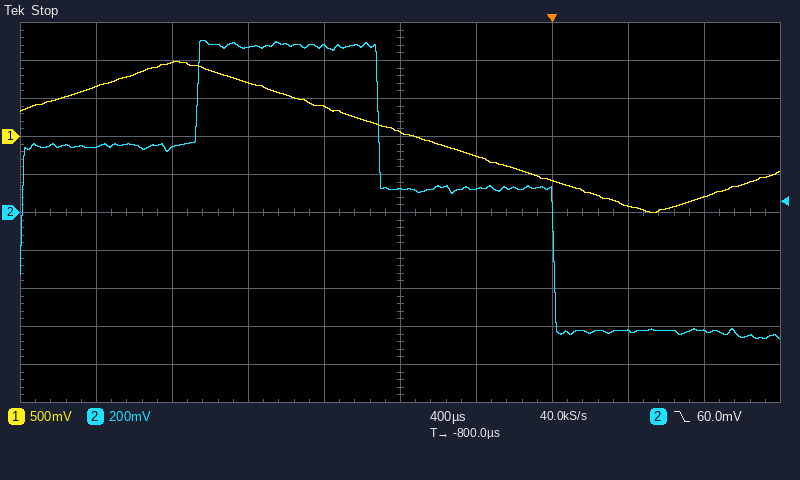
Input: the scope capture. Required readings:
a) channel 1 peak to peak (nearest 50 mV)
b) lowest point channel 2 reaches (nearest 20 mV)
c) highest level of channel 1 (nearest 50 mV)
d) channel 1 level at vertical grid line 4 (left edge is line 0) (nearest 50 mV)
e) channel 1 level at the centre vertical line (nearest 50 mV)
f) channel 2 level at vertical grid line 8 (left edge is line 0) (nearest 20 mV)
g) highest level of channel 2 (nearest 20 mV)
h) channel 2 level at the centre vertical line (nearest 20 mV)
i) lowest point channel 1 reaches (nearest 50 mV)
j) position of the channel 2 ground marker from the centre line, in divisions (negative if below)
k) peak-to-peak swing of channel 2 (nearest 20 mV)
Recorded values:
2.00 V
-660 mV
1.00 V
400 mV
50 mV
-620 mV
900 mV
120 mV
-1.00 V
0.0 div
1.56 V
